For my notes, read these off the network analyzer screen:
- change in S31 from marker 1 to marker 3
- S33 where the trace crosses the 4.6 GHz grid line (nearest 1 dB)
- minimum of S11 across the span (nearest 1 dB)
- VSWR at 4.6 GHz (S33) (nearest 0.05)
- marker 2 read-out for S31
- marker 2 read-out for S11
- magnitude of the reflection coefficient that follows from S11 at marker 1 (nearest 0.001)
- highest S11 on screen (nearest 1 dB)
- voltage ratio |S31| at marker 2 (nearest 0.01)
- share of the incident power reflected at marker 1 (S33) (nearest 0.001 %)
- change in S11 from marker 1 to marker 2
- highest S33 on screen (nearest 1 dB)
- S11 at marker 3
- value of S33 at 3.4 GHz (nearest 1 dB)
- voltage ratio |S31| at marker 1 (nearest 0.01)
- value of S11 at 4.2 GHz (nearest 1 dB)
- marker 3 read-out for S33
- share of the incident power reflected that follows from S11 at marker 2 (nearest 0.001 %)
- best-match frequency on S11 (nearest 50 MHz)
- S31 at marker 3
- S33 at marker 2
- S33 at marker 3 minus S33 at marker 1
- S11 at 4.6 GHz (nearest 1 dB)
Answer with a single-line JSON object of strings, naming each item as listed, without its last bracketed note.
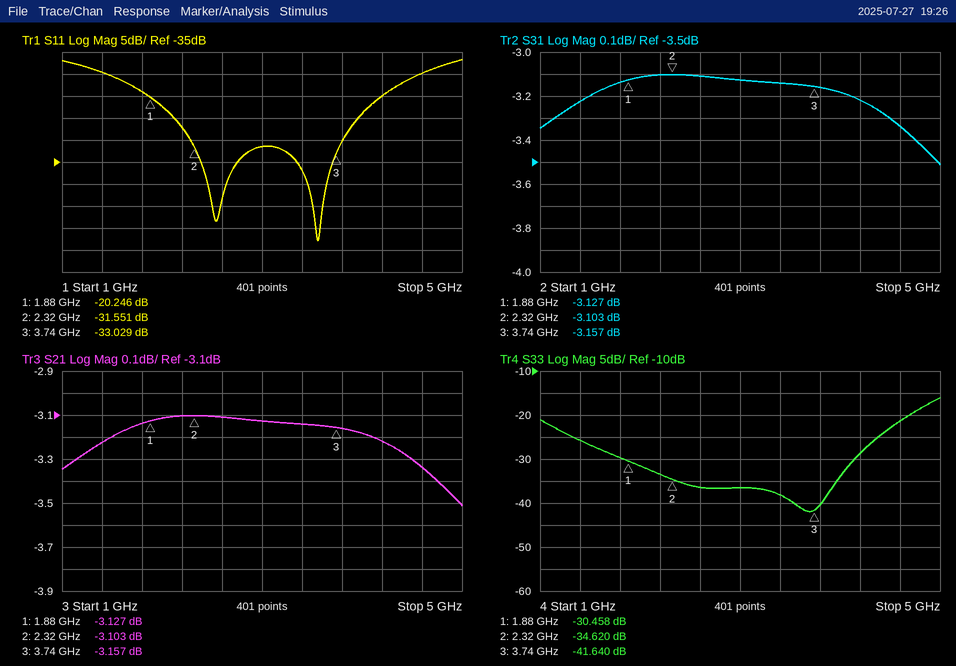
{"change in S31 from marker 1 to marker 3": "-0.030 dB", "S33 where the trace crosses the 4.6 GHz grid line": "-21 dB", "minimum of S11 across the span": "-53 dB", "VSWR at 4.6 GHz (S33)": "1.20", "marker 2 read-out for S31": "-3.103 dB", "marker 2 read-out for S11": "-31.551 dB", "magnitude of the reflection coefficient that follows from S11 at marker 1": "0.097", "highest S11 on screen": "-12 dB", "voltage ratio |S31| at marker 2": "0.70", "share of the incident power reflected at marker 1 (S33)": "0.090 %", "change in S11 from marker 1 to marker 2": "-11.305 dB", "highest S33 on screen": "-16 dB", "S11 at marker 3": "-33.029 dB", "value of S33 at 3.4 GHz": "-38 dB", "voltage ratio |S31| at marker 1": "0.70", "value of S11 at 4.2 GHz": "-20 dB", "marker 3 read-out for S33": "-41.640 dB", "share of the incident power reflected that follows from S11 at marker 2": "0.070 %", "best-match frequency on S11": "3.55 GHz", "S31 at marker 3": "-3.157 dB", "S33 at marker 2": "-34.620 dB", "S33 at marker 3 minus S33 at marker 1": "-11.182 dB", "S11 at 4.6 GHz": "-15 dB"}
